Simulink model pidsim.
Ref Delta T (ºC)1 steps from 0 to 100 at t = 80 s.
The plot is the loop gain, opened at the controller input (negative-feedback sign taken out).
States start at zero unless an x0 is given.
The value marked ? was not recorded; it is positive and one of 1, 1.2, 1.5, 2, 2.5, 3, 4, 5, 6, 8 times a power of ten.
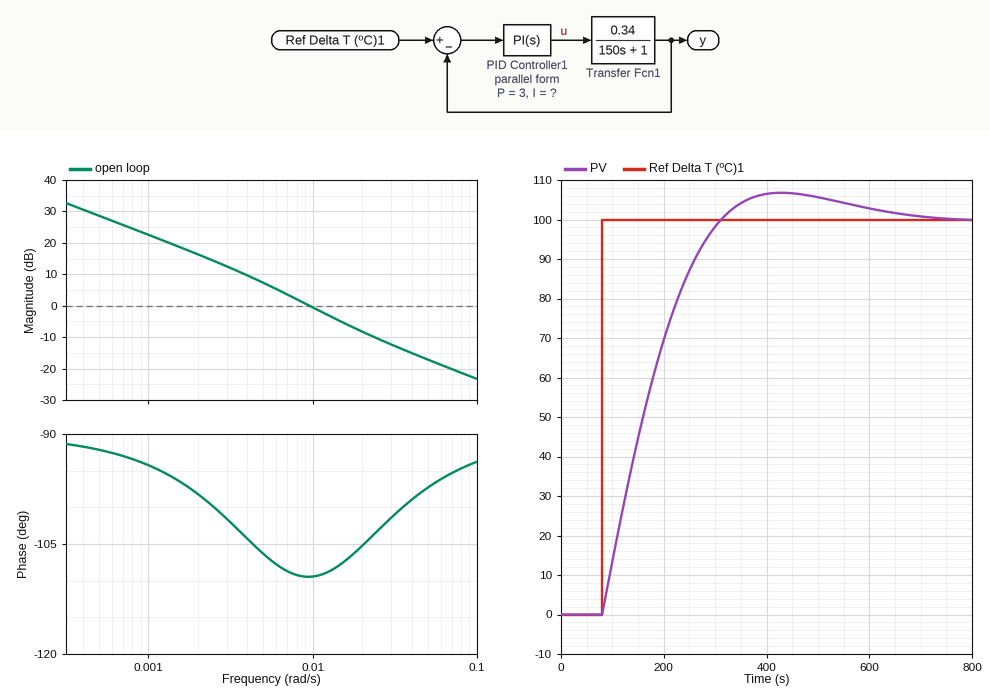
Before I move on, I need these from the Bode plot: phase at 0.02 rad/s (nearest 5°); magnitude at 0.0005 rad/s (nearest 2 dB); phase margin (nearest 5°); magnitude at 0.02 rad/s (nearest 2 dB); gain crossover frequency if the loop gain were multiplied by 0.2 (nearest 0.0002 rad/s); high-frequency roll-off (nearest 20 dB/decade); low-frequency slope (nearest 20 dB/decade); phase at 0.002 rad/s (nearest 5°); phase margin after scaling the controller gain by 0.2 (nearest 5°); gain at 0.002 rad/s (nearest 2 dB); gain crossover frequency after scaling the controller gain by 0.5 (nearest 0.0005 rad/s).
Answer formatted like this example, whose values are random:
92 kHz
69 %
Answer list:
-105°
28 dB
70°
-8 dB
0.0026 rad/s
-20 dB/decade
-20 dB/decade
-100°
80°
16 dB
0.0055 rad/s
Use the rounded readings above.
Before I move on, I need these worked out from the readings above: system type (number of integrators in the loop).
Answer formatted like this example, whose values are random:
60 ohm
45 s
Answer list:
1
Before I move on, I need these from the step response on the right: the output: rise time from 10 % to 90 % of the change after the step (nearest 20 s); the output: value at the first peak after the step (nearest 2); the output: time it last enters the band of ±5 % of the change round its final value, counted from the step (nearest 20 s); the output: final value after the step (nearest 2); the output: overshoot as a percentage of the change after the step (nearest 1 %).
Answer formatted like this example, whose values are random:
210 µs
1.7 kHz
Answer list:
160 s
106
440 s
100
7 %
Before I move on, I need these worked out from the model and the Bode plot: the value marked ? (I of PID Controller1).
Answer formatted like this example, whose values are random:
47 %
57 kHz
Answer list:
0.04
